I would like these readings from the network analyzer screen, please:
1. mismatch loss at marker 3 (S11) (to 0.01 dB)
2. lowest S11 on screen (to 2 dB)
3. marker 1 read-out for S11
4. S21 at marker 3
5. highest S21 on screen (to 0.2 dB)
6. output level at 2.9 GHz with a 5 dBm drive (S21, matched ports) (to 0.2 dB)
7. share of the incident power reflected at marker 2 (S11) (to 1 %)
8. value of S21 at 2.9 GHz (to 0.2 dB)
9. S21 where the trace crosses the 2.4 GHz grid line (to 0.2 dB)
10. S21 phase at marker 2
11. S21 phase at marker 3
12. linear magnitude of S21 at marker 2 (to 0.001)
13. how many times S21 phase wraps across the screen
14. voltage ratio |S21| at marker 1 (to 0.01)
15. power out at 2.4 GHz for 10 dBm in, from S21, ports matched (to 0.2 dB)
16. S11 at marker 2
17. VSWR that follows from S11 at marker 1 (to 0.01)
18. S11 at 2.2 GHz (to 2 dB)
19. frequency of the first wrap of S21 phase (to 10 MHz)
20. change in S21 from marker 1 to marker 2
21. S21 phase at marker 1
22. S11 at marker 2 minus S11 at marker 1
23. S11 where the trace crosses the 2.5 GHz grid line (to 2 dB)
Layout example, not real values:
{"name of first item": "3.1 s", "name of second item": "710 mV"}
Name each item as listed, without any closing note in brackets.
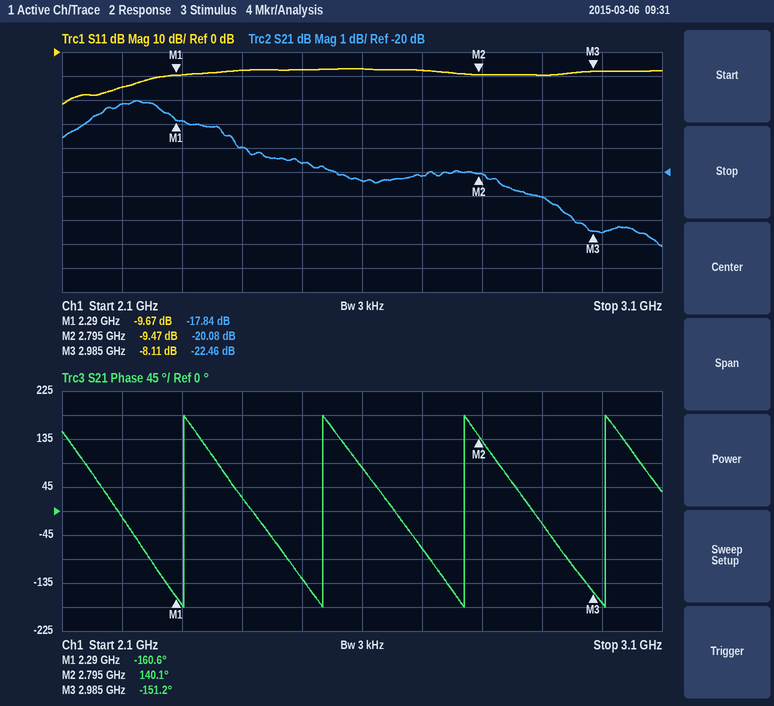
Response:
{"mismatch loss at marker 3 (S11)": "0.73 dB", "lowest S11 on screen": "-22 dB", "marker 1 read-out for S11": "-9.67 dB", "S21 at marker 3": "-22.46 dB", "highest S21 on screen": "-17.0 dB", "output level at 2.9 GHz with a 5 dBm drive (S21, matched ports)": "-16.0 dBm", "share of the incident power reflected at marker 2 (S11)": "11 %", "value of S21 at 2.9 GHz": "-21.0 dB", "S21 where the trace crosses the 2.4 GHz grid line": "-19.0 dB", "S21 phase at marker 2": "140.1°", "S21 phase at marker 3": "-151.2°", "linear magnitude of S21 at marker 2": "0.099", "how many times S21 phase wraps across the screen": "4", "voltage ratio |S21| at marker 1": "0.13", "power out at 2.4 GHz for 10 dBm in, from S21, ports matched": "-9.0 dBm", "S11 at marker 2": "-9.47 dB", "VSWR that follows from S11 at marker 1": "1.98", "S11 at 2.2 GHz": "-14 dB", "frequency of the first wrap of S21 phase": "2.30 GHz", "change in S21 from marker 1 to marker 2": "-2.24 dB", "S21 phase at marker 1": "-160.6°", "S11 at marker 2 minus S11 at marker 1": "0.20 dB", "S11 where the trace crosses the 2.5 GHz grid line": "-8 dB"}
